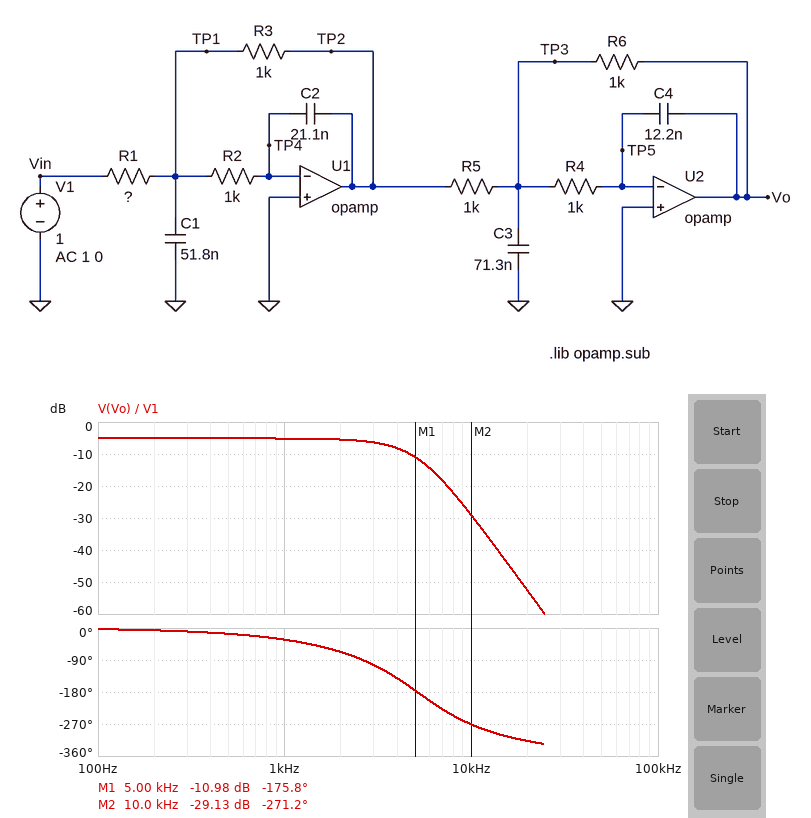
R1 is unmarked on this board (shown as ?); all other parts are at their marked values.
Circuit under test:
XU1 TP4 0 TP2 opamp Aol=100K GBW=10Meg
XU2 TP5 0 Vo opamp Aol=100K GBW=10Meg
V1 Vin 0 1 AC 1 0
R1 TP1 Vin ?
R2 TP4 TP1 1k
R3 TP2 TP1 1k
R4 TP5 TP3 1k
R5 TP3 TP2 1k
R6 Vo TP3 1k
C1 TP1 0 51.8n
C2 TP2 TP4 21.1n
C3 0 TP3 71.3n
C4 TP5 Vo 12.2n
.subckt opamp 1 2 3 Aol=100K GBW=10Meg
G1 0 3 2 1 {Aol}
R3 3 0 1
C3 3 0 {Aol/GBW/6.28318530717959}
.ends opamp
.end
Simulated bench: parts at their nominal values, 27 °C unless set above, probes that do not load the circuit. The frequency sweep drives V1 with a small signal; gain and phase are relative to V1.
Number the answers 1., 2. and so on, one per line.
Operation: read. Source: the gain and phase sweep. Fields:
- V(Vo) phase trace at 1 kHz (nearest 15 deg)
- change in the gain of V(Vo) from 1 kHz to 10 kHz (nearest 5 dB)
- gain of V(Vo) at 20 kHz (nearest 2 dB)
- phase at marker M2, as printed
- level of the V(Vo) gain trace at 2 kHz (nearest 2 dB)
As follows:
1. -30 deg
2. -25 dB
3. -52 dB
4. -271.2 deg
5. -6 dB
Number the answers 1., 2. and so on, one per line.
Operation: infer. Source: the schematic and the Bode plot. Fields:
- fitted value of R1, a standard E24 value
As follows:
1. 1.8 kΩ
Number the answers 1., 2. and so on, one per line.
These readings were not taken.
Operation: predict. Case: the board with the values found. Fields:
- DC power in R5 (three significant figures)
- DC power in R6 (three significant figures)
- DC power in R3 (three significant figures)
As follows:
1. 309 µW
2. 309 µW
3. 309 µW
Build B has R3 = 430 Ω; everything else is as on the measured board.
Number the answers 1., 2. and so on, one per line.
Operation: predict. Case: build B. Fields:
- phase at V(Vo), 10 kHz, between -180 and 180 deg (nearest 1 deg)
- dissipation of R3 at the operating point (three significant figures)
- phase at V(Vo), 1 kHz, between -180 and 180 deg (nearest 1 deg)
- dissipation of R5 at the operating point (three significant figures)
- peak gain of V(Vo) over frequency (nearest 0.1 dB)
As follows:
1. 112 deg
2. 133 µW
3. -26 deg
4. 57.1 µW
5. -12.4 dB
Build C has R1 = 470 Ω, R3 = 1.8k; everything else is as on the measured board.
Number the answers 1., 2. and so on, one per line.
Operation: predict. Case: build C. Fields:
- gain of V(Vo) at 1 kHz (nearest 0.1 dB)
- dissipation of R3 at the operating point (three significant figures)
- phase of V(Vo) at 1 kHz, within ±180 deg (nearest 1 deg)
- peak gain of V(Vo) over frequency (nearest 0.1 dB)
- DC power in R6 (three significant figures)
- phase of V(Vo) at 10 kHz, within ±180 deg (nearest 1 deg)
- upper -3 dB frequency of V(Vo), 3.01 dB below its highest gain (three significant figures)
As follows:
1. 9.6 dB
2. 8.15 mW
3. -57 deg
4. 11.7 dB
5. 14.7 mW
6. 96 deg
7. 1.29 kHz
